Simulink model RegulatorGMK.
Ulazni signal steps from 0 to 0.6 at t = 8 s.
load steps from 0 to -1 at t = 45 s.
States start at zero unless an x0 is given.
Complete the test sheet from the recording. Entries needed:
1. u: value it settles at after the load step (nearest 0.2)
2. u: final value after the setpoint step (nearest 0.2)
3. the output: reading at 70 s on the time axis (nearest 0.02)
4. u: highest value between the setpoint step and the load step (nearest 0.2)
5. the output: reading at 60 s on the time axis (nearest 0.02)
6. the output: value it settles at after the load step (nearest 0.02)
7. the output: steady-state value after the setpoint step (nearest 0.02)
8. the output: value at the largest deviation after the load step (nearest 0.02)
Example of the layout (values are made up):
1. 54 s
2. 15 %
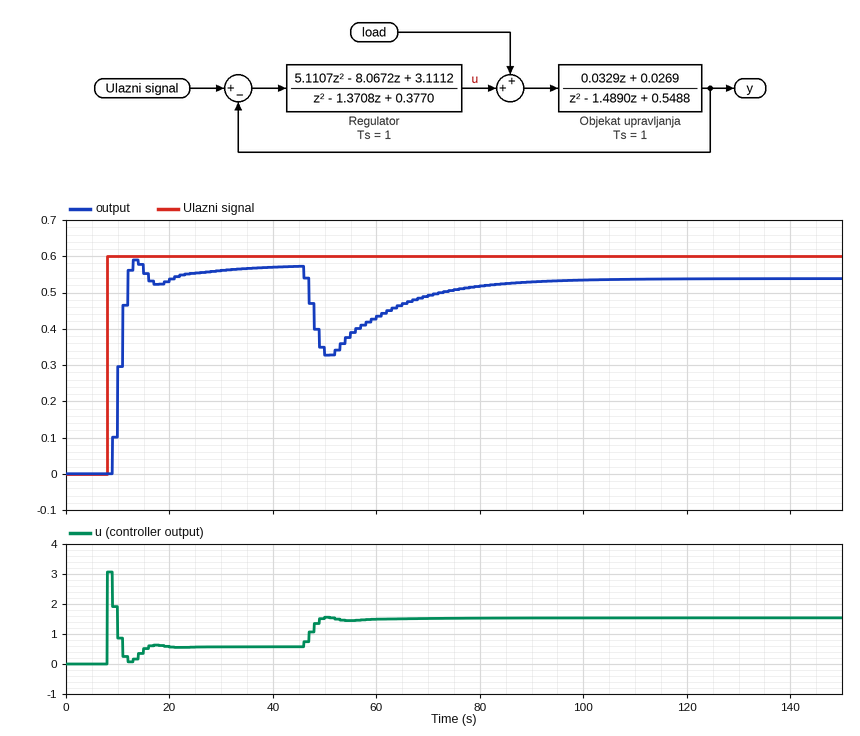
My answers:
1. 1.6
2. 0.6
3. 0.50
4. 3.0
5. 0.44
6. 0.54
7. 0.58
8. 0.32
